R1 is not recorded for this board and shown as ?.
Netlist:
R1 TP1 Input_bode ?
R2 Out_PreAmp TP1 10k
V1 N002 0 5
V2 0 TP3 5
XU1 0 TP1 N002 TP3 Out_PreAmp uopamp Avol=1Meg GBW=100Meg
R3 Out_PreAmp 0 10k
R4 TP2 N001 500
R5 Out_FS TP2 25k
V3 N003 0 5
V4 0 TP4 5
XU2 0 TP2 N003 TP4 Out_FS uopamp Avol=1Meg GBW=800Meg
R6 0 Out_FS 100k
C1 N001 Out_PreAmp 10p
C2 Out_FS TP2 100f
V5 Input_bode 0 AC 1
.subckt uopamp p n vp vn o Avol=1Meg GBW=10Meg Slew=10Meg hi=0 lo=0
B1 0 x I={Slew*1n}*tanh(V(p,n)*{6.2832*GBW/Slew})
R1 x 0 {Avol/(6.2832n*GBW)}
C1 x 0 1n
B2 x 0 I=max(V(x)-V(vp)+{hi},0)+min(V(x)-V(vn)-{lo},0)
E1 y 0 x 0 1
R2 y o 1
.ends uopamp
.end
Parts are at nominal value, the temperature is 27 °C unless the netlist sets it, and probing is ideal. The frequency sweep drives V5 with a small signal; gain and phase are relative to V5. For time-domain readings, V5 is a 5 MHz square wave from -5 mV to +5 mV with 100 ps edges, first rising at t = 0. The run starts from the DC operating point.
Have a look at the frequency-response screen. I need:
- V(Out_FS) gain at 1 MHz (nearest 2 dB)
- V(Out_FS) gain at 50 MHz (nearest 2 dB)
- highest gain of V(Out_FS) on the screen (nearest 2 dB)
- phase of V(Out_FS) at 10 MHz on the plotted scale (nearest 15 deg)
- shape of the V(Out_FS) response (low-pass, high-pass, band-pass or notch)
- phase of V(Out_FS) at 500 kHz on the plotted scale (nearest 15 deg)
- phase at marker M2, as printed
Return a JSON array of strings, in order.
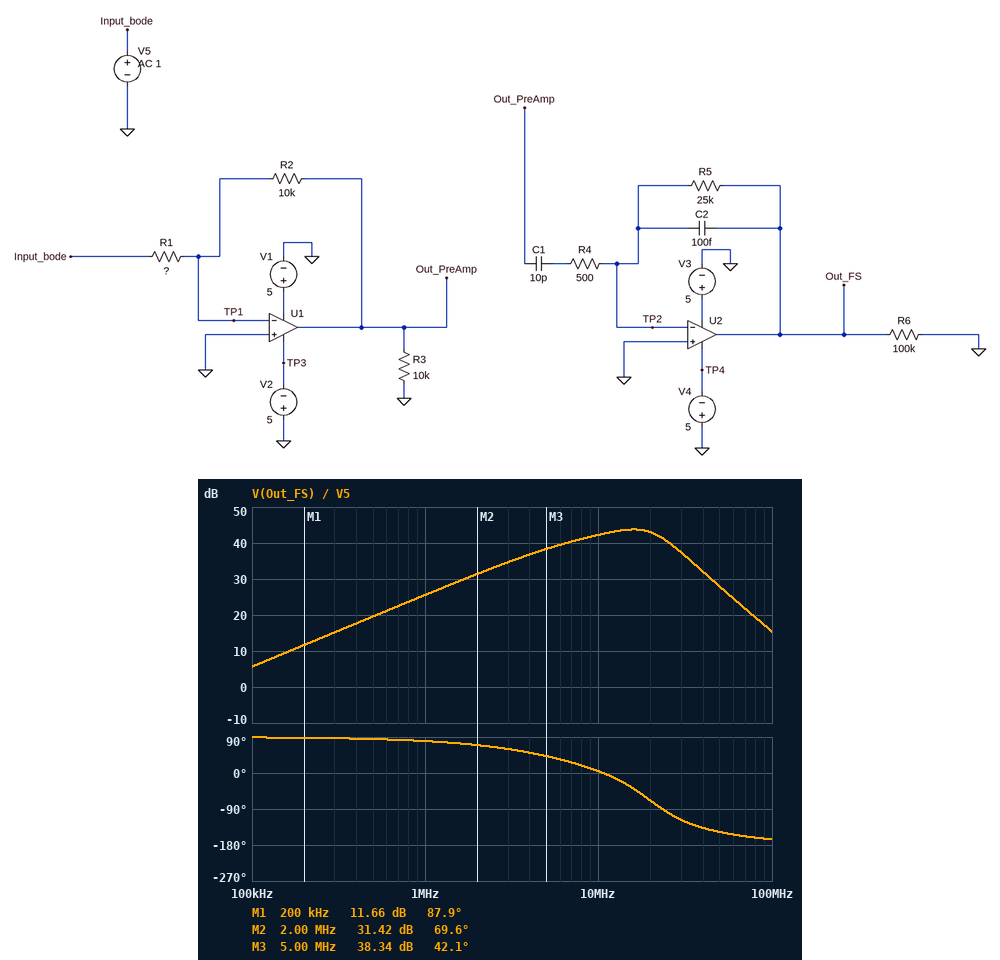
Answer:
["26 dB", "28 dB", "44 dB", "0 deg", "band-pass", "90 deg", "69.6 deg"]
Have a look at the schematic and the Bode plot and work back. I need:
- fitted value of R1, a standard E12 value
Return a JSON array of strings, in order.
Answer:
["820 Ω"]
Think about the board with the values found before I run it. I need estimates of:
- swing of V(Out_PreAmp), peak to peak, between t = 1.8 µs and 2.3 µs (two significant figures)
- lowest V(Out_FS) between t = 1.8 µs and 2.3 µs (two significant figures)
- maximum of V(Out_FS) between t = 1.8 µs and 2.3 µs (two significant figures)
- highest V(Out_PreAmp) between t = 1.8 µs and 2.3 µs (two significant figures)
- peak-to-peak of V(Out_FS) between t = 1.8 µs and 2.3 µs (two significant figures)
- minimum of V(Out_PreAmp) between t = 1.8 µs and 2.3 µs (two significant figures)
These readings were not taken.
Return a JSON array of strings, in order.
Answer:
["120 mV", "-500 mV", "500 mV", "60 mV", "1.0 V", "-60 mV"]
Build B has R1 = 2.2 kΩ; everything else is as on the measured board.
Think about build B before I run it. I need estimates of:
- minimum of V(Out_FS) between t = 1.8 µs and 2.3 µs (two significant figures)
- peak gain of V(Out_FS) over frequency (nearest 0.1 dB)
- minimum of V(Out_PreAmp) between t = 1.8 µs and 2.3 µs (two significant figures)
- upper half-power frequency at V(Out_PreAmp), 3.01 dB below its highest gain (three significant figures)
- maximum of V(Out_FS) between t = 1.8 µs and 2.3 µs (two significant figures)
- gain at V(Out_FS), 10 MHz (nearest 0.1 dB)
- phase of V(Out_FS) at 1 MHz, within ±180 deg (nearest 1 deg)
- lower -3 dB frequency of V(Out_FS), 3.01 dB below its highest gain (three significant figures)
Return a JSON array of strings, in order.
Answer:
["-490 mV", "40.2 dB", "-23 mV", "18.0 MHz", "490 mV", "36.9 dB", "84 deg", "10.4 MHz"]
